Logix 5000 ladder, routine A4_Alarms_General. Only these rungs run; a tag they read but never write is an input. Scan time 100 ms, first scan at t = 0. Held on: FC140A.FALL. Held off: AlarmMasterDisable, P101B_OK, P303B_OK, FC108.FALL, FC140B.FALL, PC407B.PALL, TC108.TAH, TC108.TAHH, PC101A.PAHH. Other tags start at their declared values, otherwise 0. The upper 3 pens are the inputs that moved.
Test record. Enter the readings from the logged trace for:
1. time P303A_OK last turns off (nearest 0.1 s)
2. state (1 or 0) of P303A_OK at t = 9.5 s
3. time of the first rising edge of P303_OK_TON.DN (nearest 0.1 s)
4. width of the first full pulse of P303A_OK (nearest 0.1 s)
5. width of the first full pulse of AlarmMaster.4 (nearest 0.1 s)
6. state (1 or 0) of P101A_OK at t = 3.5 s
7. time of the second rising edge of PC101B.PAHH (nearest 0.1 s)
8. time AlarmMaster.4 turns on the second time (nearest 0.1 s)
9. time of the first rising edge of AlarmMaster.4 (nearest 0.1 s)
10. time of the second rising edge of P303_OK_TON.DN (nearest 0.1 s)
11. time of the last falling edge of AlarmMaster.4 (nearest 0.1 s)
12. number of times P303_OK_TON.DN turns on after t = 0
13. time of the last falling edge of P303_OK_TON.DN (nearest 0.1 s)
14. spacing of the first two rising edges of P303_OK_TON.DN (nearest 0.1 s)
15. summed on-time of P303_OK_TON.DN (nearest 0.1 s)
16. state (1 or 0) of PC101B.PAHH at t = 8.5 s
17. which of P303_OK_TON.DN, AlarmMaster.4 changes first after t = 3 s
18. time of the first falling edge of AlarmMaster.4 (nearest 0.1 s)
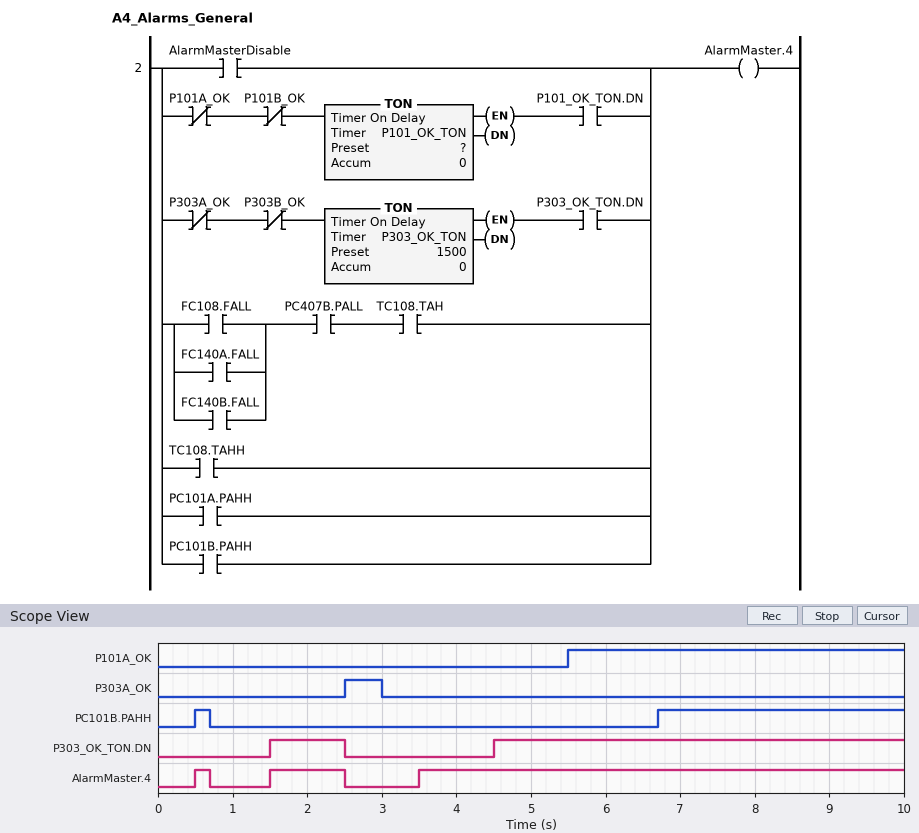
3.0 s
0
1.5 s
0.5 s
0.2 s
0
6.7 s
1.5 s
0.5 s
4.5 s
2.5 s
2
2.5 s
3.0 s
6.5 s
1
AlarmMaster.4
0.7 s
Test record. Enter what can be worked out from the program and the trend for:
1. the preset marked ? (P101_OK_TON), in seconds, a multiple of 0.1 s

3.5 s
